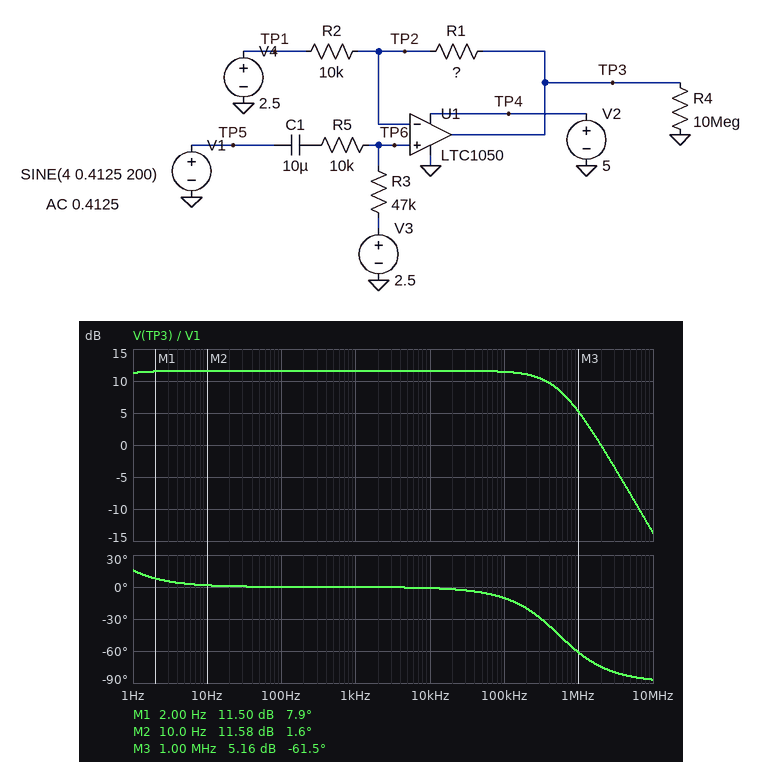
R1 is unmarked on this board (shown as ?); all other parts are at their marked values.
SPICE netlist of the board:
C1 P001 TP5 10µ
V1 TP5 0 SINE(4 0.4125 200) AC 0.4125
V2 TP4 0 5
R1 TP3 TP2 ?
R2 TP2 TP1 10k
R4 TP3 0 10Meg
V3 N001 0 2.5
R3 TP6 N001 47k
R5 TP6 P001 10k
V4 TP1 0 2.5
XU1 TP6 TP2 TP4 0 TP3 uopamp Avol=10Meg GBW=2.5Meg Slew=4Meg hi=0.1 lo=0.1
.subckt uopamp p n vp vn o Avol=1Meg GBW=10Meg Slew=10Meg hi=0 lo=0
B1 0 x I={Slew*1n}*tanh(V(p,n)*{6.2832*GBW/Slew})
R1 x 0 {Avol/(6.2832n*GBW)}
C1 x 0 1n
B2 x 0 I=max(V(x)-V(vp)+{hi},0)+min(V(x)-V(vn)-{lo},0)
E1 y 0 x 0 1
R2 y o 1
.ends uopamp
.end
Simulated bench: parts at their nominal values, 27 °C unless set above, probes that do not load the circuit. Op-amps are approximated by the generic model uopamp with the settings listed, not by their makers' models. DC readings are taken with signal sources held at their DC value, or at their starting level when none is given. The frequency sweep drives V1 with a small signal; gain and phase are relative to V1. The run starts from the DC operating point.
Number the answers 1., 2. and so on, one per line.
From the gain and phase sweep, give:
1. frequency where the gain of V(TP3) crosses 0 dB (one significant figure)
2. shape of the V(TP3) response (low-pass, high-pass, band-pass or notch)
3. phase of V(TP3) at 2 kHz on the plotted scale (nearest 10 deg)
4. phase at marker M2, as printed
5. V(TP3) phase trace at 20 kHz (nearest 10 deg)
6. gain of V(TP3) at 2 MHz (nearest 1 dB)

1. 2 MHz
2. low-pass
3. 0 deg
4. 1.6 deg
5. 0 deg
6. 0 dB
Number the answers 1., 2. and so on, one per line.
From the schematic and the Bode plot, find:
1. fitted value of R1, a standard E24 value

1. 36 kΩ
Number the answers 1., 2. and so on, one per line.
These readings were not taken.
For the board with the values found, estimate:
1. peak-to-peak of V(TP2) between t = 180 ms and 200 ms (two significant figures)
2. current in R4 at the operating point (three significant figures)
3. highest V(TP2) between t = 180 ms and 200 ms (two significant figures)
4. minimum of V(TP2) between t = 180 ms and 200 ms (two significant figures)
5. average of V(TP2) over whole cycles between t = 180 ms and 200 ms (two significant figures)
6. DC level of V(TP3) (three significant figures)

1. 680 mV
2. 250 nA
3. 2.8 V
4. 2.2 V
5. 2.5 V
6. 2.50 V
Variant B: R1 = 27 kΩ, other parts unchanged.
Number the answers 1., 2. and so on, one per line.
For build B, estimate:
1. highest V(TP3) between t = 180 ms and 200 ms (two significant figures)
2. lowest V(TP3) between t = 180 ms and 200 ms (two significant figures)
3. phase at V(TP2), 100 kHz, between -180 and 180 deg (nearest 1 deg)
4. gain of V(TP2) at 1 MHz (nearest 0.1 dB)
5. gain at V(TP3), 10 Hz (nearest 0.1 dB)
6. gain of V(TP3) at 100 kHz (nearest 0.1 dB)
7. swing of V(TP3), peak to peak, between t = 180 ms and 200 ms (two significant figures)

1. 3.8 V
2. 1.2 V
3. -8 deg
4. -6.7 dB
5. 9.7 dB
6. 9.6 dB
7. 2.5 V
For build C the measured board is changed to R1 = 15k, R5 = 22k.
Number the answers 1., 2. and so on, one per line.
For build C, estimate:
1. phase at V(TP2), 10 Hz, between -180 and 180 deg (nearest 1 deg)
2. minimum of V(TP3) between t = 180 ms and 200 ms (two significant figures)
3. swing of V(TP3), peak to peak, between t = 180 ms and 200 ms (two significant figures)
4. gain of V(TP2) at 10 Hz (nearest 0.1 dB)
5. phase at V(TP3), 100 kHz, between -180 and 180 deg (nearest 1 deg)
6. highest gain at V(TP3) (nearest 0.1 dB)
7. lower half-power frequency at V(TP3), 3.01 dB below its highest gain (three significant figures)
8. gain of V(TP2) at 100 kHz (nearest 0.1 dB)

1. 1 deg
2. 1.8 V
3. 1.4 V
4. -3.3 dB
5. -6 deg
6. 4.6 dB
7. 231 mHz
8. -3.4 dB
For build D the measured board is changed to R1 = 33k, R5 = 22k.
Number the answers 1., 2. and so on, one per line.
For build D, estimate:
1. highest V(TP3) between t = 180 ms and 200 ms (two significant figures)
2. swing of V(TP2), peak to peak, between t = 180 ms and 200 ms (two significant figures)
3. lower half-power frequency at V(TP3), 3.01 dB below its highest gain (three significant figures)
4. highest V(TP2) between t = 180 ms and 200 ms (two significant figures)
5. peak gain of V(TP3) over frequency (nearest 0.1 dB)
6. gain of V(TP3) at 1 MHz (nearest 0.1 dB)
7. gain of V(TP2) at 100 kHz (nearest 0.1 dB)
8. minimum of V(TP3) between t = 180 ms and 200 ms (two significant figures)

1. 3.7 V
2. 560 mV
3. 231 mHz
4. 2.8 V
5. 9.3 dB
6. 3.4 dB
7. -3.5 dB
8. 1.3 V
